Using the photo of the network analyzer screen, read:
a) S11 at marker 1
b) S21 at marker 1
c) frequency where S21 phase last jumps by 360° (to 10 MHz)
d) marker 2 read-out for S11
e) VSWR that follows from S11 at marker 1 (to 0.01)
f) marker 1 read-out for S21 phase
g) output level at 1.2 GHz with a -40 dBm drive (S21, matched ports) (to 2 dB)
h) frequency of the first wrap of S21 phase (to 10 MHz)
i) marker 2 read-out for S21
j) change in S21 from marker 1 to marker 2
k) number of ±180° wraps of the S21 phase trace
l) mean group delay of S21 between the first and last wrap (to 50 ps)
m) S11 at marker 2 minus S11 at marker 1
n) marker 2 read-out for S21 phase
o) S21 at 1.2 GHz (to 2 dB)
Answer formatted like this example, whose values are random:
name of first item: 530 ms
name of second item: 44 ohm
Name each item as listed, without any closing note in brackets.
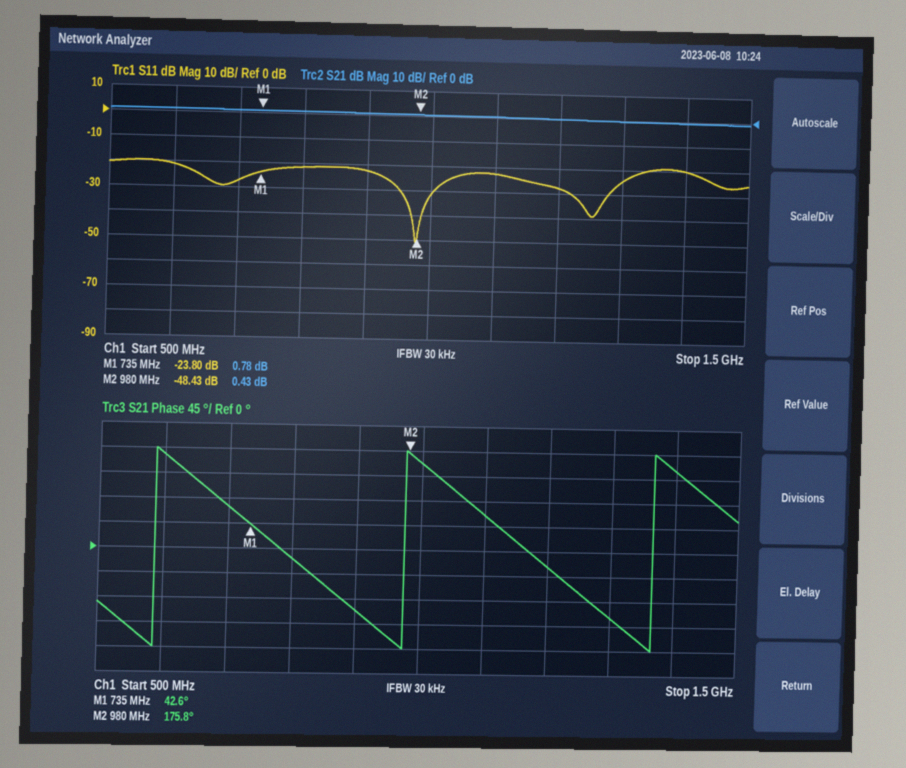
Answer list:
S11 at marker 1: -23.80 dB
S21 at marker 1: 0.78 dB
frequency where S21 phase last jumps by 360°: 1.37 GHz
marker 2 read-out for S11: -48.43 dB
VSWR that follows from S11 at marker 1: 1.14
marker 1 read-out for S21 phase: 42.6°
output level at 1.2 GHz with a -40 dBm drive (S21, matched ports): -40 dBm
frequency of the first wrap of S21 phase: 590 MHz
marker 2 read-out for S21: 0.43 dB
change in S21 from marker 1 to marker 2: -0.35 dB
number of ±180° wraps of the S21 phase trace: 3
mean group delay of S21 between the first and last wrap: 2.55 ns
S11 at marker 2 minus S11 at marker 1: -24.63 dB
marker 2 read-out for S21 phase: 175.8°
S21 at 1.2 GHz: 0 dB
